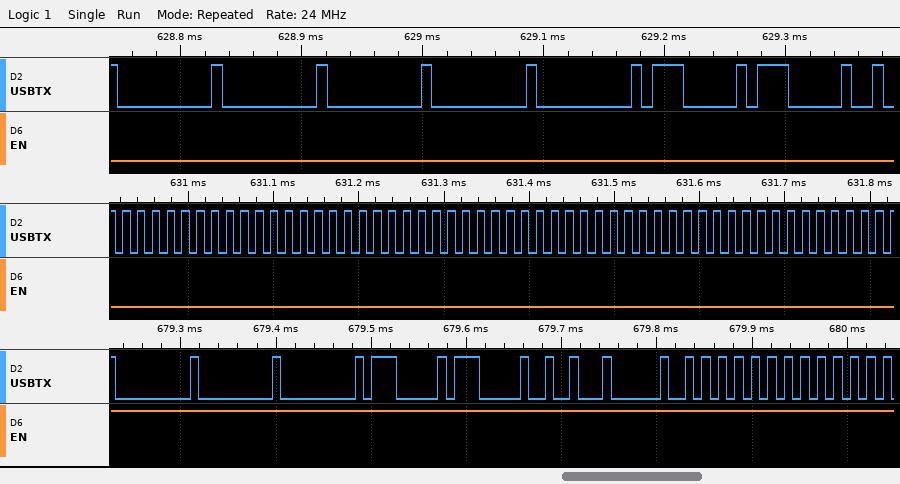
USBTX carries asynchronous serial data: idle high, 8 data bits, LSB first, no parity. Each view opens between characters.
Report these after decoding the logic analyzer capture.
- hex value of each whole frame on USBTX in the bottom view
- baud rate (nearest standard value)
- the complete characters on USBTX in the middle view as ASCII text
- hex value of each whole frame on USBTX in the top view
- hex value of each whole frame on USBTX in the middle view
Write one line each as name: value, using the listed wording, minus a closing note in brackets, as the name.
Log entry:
hex value of each whole frame on USBTX in the bottom view: 00, 00, 00, 07, 07, 12, 20, 55, 55
baud rate: 115200 baud
the complete characters on USBTX in the middle view as ASCII text: "UUUUUUUUUU"
hex value of each whole frame on USBTX in the top view: 00, 00, 00, 00, 00, 07, 07
hex value of each whole frame on USBTX in the middle view: 55, 55, 55, 55, 55, 55, 55, 55, 55, 55
